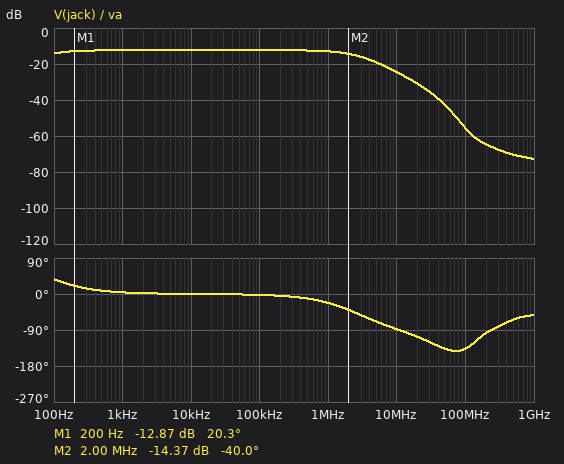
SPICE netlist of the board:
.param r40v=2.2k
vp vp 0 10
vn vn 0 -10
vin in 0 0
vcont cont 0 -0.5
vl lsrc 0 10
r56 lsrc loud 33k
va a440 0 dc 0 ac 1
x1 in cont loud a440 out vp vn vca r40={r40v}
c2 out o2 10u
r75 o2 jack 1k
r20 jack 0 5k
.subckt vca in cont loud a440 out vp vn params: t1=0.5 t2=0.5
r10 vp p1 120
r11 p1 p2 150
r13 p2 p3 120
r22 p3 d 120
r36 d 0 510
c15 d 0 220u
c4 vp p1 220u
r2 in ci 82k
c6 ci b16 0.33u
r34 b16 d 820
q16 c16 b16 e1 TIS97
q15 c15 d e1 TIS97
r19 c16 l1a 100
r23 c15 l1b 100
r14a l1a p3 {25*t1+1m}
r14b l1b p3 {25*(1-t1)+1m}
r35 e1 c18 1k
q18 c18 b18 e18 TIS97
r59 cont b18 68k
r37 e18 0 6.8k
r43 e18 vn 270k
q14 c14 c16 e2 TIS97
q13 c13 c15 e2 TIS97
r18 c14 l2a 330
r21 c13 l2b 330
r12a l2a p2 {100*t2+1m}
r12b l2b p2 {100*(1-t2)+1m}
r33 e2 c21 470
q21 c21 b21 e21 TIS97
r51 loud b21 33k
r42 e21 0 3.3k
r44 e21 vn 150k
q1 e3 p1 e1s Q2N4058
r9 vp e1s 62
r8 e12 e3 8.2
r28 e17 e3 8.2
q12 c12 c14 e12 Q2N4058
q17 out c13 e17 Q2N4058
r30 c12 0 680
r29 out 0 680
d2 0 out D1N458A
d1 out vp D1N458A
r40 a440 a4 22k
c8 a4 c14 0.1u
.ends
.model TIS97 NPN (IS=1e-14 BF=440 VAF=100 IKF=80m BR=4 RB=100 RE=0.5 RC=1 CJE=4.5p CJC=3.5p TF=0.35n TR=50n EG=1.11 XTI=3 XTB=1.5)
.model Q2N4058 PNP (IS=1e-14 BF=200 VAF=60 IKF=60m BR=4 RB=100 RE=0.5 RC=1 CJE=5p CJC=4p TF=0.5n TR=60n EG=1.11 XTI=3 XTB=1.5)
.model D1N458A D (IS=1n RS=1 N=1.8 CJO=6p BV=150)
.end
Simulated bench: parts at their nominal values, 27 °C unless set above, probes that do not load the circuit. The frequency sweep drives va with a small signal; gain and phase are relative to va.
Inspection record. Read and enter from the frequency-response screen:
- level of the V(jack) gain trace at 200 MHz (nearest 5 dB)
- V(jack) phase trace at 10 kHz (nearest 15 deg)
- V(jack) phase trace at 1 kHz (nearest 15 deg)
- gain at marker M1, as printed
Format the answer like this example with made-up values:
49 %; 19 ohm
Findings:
-65 dB; 0 deg; 0 deg; -12.87 dB
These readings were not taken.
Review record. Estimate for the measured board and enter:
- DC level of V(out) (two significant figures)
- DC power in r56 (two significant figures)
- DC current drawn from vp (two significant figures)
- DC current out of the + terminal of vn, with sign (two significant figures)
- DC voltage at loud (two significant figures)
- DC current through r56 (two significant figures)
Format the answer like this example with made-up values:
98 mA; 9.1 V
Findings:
3.1 V; 170 µW; 20 mA; -130 µA; 7.6 V; 72 µA
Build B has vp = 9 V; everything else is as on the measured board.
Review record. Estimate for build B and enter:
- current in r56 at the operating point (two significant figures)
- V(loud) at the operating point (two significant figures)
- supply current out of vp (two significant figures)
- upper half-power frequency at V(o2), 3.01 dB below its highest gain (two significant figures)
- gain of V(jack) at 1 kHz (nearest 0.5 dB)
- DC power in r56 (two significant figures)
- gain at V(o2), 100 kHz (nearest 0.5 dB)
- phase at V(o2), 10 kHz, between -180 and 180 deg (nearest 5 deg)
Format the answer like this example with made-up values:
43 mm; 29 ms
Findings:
79 µA; 7.4 V; 17 mA; 2.8 MHz; -13.0 dB; 210 µW; -11.5 dB; 0 deg
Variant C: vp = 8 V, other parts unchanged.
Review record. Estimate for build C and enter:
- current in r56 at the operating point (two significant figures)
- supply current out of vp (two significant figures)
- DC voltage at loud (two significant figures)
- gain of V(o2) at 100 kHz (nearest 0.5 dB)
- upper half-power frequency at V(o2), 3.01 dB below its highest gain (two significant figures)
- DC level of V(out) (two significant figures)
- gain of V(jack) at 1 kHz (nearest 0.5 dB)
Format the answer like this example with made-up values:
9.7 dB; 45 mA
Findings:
87 µA; 14 mA; 7.1 V; -12.5 dB; 3.1 MHz; 1.8 V; -14.0 dB
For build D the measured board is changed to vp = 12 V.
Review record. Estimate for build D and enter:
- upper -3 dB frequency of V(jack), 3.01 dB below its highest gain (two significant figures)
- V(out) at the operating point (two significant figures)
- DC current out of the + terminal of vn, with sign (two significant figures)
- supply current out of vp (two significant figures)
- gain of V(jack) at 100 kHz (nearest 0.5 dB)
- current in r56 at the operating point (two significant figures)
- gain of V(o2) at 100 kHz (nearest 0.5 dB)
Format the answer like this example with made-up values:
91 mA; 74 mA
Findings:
2.4 MHz; 4.4 V; -140 µA; 26 mA; -11.5 dB; 56 µA; -10.0 dB
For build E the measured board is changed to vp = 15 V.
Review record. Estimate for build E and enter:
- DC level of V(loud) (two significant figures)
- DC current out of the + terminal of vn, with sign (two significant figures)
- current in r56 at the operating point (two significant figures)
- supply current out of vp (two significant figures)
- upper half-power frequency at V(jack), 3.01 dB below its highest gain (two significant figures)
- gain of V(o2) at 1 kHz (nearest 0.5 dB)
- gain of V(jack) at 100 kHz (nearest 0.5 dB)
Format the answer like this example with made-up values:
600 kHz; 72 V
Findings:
8.9 V; -150 µA; 33 µA; 35 mA; 2.3 MHz; -9.5 dB; -11.0 dB
